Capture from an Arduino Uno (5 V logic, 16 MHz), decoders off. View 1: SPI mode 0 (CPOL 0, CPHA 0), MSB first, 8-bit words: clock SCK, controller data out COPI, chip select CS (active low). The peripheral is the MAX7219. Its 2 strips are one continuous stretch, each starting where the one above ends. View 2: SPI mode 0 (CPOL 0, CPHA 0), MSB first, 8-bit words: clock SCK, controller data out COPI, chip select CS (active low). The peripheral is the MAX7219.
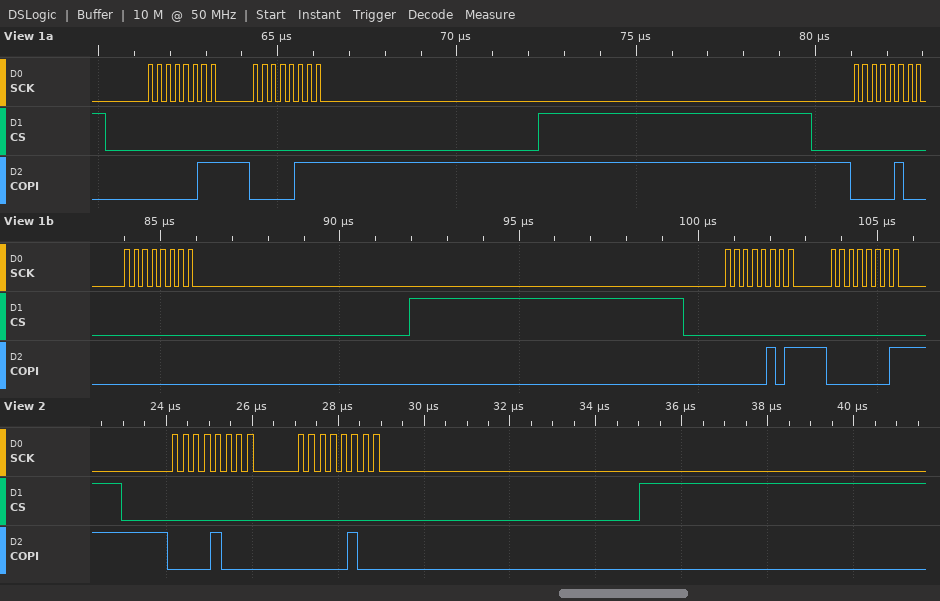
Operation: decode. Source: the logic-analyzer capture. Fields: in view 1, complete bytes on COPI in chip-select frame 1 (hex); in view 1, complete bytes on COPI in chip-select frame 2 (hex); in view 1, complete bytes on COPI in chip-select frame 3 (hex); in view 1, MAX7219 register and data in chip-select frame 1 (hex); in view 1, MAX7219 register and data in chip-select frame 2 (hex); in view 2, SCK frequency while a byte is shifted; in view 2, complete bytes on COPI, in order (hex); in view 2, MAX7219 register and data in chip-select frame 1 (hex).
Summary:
0x03 0x07
0x04 0x00
0x05 0x01
register 0x3, data 0x07
register 0x4, data 0x00
4 MHz
08 04
register 0x8, data 0x04
